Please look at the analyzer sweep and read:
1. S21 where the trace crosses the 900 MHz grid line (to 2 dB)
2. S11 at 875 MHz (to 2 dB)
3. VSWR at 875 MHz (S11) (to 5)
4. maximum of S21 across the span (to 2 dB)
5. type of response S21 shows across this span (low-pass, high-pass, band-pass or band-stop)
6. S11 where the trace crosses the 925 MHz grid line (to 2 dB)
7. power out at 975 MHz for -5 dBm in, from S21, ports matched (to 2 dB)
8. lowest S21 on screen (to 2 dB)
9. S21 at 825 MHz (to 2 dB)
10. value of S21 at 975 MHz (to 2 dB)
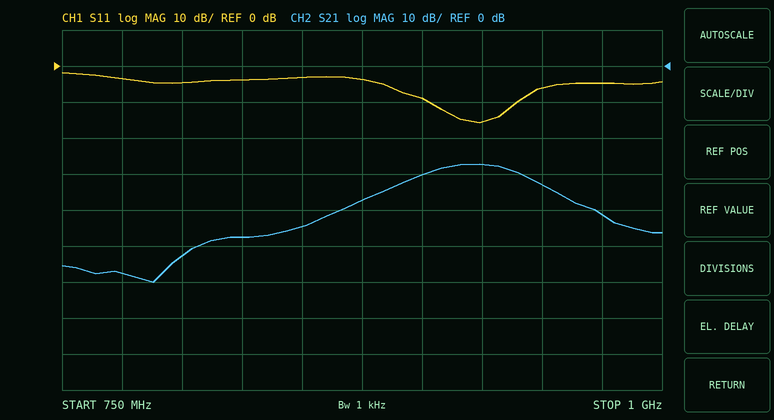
-30 dB
-4 dB
5
-28 dB
band-pass
-16 dB
-46 dBm
-60 dB
-48 dB
-42 dB
